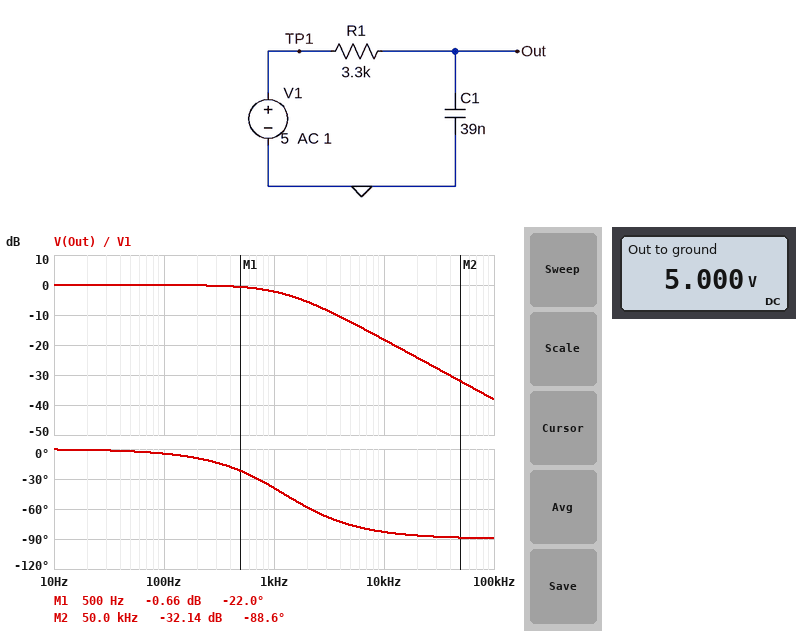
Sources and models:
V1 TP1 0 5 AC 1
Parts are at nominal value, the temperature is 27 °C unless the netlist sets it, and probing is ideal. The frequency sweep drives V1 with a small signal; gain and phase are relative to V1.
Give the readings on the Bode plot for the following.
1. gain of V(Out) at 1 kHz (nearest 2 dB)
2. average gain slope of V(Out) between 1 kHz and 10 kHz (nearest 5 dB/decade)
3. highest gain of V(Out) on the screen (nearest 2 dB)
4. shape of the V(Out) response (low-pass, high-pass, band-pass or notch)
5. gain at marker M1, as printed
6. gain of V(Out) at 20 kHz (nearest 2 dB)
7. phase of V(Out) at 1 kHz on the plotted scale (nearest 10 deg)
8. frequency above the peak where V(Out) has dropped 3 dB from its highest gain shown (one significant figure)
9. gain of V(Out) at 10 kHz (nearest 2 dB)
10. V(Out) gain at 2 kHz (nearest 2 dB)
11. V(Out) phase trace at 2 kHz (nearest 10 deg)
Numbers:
-2 dB
-15 dB/decade
0 dB
low-pass
-0.66 dB
-24 dB
-40 deg
1 kHz
-18 dB
-6 dB
-60 deg
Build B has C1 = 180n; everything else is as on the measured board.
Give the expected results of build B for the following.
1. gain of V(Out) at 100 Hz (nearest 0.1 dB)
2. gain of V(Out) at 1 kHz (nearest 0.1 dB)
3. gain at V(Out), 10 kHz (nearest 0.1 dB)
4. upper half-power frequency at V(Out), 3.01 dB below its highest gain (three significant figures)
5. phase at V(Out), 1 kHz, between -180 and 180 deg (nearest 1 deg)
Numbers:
-0.6 dB
-11.7 dB
-31.4 dB
268 Hz
-75 deg
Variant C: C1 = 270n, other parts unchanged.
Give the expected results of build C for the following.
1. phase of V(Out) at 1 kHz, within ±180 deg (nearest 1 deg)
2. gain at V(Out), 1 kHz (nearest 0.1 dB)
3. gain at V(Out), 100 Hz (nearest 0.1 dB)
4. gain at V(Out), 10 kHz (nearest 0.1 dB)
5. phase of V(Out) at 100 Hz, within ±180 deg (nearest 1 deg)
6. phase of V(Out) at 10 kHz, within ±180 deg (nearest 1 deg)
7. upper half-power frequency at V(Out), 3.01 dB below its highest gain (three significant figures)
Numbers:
-80 deg
-15.1 dB
-1.2 dB
-35.0 dB
-29 deg
-89 deg
179 Hz
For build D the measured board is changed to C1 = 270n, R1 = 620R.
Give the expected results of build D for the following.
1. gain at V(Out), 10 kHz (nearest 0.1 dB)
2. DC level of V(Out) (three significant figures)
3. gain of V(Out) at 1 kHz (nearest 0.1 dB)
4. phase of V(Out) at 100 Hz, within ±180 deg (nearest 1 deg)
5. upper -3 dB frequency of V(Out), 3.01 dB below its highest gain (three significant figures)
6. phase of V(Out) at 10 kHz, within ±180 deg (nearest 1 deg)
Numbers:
-20.5 dB
5.00 V
-3.2 dB
-6 deg
951 Hz
-85 deg
